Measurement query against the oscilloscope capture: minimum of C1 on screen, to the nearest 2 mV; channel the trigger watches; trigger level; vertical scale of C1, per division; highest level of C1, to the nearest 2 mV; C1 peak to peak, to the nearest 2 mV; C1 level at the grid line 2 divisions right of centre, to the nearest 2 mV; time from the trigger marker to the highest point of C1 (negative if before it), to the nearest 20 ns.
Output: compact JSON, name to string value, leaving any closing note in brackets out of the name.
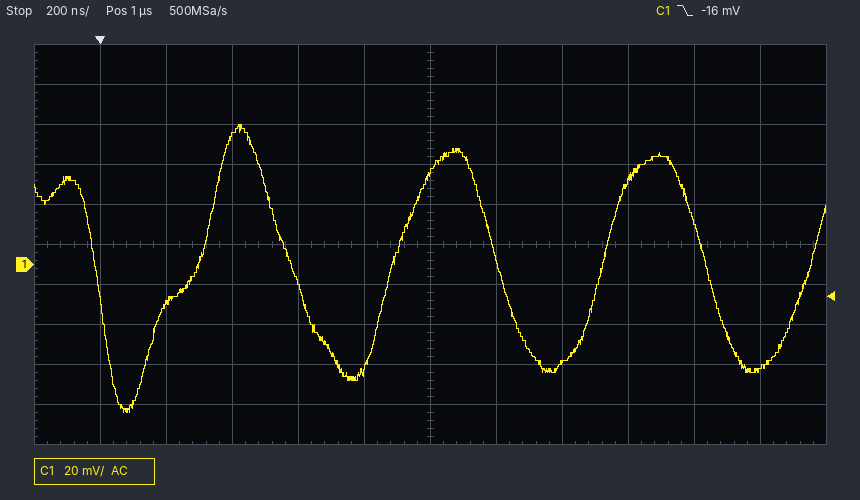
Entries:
{"minimum of C1 on screen, to the nearest 2 mV": "-74 mV", "channel the trigger watches": "C1", "trigger level": "-16 mV", "vertical scale of C1, per division": "20 mV", "highest level of C1, to the nearest 2 mV": "70 mV", "C1 peak to peak, to the nearest 2 mV": "144 mV", "C1 level at the grid line 2 divisions right of centre, to the nearest 2 mV": "-48 mV", "time from the trigger marker to the highest point of C1 (negative if before it), to the nearest 20 ns": "+420 ns"}
